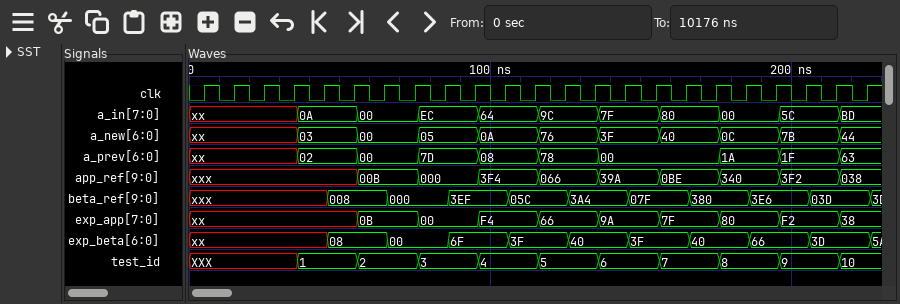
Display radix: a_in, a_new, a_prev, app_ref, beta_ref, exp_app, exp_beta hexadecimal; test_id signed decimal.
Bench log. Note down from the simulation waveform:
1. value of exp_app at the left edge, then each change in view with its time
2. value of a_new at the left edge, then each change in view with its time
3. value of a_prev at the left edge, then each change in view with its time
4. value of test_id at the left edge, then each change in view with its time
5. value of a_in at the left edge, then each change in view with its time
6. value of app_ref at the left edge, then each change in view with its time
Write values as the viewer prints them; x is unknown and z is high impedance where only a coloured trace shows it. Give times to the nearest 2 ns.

xx, 0B at 56 ns, 00 at 76 ns, F4 at 96 ns, 66 at 116 ns, 9A at 136 ns, 7F at 156 ns, 80 at 176 ns, F2 at 196 ns, 38 at 216 ns
xx, 03 at 36 ns, 00 at 56 ns, 05 at 76 ns, 0A at 96 ns, 76 at 116 ns, 3F at 136 ns, 40 at 156 ns, 0C at 176 ns, 7B at 196 ns, 44 at 216 ns
xx, 02 at 36 ns, 00 at 56 ns, 7D at 76 ns, 08 at 96 ns, 78 at 116 ns, 00 at 136 ns, 1A at 176 ns, 1F at 196 ns, 63 at 216 ns
XXX, 1 at 36 ns, 2 at 56 ns, 3 at 76 ns, 4 at 96 ns, 5 at 116 ns, 6 at 136 ns, 7 at 156 ns, 8 at 176 ns, 9 at 196 ns, 10 at 216 ns
xx, 0A at 36 ns, 00 at 56 ns, EC at 76 ns, 64 at 96 ns, 9C at 116 ns, 7F at 136 ns, 80 at 156 ns, 00 at 176 ns, 5C at 196 ns, BD at 216 ns
xxx, 00B at 56 ns, 000 at 76 ns, 3F4 at 96 ns, 066 at 116 ns, 39A at 136 ns, 0BE at 156 ns, 340 at 176 ns, 3F2 at 196 ns, 038 at 216 ns
